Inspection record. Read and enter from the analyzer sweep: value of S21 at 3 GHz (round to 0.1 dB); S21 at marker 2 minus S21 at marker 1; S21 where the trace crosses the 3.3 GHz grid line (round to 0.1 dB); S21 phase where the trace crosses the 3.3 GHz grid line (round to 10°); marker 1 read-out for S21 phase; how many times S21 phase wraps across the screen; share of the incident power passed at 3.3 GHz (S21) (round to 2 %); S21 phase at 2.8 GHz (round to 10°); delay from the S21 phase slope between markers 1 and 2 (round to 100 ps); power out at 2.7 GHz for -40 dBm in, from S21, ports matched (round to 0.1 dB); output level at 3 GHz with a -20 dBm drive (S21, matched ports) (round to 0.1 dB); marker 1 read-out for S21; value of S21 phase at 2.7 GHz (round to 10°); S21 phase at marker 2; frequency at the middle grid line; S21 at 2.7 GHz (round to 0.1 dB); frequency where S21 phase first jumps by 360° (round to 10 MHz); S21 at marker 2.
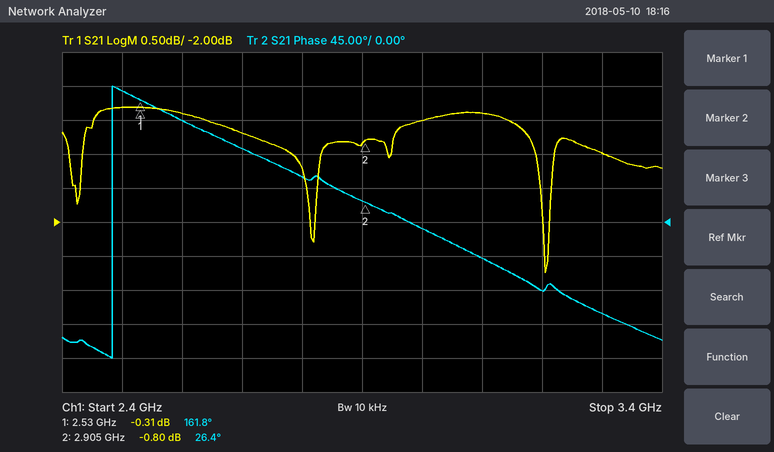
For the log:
-0.5 dB
-0.49 dB
-1.0 dB
-120°
161.8°
1
80 %
60°
1.0 ns
-40.7 dBm
-20.5 dBm
-0.31 dB
100°
26.4°
2.9 GHz
-0.7 dB
2.48 GHz
-0.80 dB
